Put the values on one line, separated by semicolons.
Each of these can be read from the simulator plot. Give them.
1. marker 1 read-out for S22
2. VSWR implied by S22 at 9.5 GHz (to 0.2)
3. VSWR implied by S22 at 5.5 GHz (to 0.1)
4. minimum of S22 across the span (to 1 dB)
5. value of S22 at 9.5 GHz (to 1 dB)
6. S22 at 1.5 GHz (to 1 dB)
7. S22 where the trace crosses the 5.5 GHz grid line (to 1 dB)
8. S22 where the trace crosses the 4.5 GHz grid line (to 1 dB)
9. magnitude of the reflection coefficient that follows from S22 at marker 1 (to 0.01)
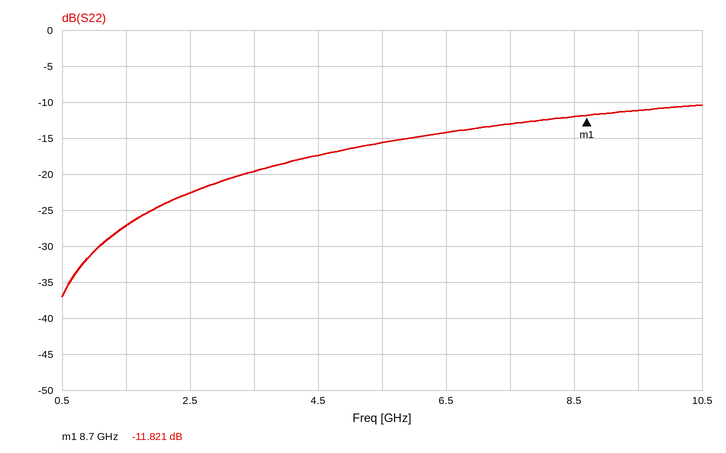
-11.821 dB; 1.8; 1.4; -37 dB; -11 dB; -27 dB; -16 dB; -17 dB; 0.26
